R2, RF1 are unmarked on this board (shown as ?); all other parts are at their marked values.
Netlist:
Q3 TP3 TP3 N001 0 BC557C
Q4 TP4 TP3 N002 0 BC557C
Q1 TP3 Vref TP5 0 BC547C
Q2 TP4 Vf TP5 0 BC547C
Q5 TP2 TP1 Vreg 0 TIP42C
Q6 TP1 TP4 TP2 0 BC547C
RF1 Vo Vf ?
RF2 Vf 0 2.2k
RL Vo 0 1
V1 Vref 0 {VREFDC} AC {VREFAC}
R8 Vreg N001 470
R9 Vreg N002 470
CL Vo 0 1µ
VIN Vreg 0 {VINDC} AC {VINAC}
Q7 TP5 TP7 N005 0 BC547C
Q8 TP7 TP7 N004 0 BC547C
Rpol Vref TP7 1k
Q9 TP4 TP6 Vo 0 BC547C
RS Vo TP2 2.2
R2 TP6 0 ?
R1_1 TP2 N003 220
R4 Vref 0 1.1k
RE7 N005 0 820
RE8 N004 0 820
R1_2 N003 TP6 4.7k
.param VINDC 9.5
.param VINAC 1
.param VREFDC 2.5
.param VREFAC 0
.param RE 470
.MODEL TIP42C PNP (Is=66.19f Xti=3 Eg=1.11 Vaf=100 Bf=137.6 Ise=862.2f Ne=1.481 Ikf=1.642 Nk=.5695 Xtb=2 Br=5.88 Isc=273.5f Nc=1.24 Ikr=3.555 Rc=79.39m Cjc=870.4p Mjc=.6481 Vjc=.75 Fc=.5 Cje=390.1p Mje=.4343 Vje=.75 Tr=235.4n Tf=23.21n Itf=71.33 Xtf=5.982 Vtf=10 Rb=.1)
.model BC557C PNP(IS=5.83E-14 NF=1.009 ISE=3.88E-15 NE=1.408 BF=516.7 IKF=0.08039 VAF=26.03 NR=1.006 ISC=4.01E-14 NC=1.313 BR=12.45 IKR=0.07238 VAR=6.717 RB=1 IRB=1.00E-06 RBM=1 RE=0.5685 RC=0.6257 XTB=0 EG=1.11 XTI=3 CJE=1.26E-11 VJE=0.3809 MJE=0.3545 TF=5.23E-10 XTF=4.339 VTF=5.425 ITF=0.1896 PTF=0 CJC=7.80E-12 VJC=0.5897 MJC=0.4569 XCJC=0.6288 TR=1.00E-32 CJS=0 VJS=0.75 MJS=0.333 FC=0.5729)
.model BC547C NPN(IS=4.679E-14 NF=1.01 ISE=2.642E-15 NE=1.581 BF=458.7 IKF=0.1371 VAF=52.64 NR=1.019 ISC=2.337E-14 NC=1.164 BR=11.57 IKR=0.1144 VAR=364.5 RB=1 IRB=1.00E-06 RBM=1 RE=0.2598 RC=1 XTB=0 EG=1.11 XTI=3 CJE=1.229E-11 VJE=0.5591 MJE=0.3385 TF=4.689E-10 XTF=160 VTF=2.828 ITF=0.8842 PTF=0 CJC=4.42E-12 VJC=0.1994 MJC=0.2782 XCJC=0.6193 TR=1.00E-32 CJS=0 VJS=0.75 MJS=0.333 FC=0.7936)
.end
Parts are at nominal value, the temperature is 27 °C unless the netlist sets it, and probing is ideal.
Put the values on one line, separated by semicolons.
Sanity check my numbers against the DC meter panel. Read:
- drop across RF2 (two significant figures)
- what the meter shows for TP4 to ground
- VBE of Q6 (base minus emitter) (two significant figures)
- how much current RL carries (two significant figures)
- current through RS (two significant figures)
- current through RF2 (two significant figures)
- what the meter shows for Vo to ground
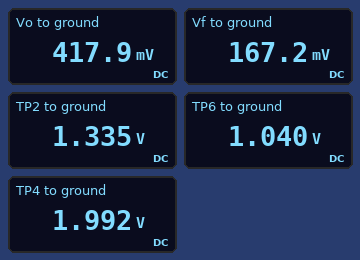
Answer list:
170 mV; 1.992 V; 660 mV; 420 mA; 420 mA; 76 µA; 417.9 mV
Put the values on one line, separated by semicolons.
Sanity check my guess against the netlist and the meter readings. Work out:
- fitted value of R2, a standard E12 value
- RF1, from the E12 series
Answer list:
18 kΩ; 3.3 kΩ
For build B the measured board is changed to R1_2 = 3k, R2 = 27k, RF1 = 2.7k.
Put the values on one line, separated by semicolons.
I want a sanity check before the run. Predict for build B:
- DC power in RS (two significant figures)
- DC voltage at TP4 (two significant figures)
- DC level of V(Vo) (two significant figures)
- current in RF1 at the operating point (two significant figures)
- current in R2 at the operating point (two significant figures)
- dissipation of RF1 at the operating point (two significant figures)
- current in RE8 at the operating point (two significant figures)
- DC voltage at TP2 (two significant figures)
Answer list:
250 mW; 1.7 V; 340 mV; 69 µA; 36 µA; 13 µW; 1.0 mA; 1.1 V
